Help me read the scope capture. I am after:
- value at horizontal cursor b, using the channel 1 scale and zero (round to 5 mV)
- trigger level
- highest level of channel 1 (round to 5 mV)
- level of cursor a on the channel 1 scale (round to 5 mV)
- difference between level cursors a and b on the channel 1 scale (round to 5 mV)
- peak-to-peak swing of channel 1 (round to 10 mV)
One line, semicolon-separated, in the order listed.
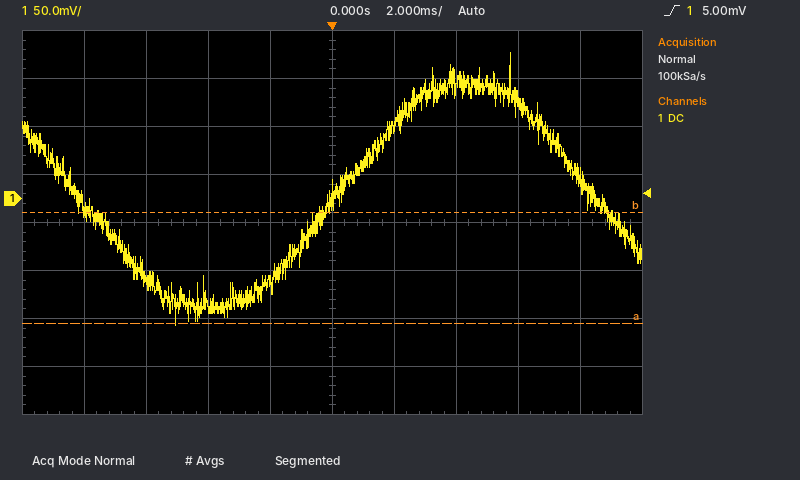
-15 mV; 5.00 mV; 150 mV; -130 mV; 115 mV; 280 mV
